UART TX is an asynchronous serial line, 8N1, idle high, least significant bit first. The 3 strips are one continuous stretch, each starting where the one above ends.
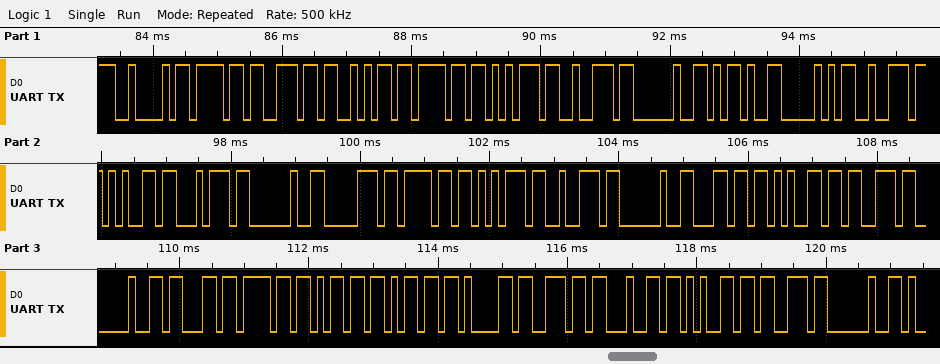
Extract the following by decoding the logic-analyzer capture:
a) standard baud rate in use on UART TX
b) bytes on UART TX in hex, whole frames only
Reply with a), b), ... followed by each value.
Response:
a) 9600 baud
b) 42 6F 6E 6A 6F 75 72 20 2D 50 72 65 74 20 70 6F 75 72 20 6C 65 73 20 63 6F 6D 6D 61 6E 64 65 73 20
